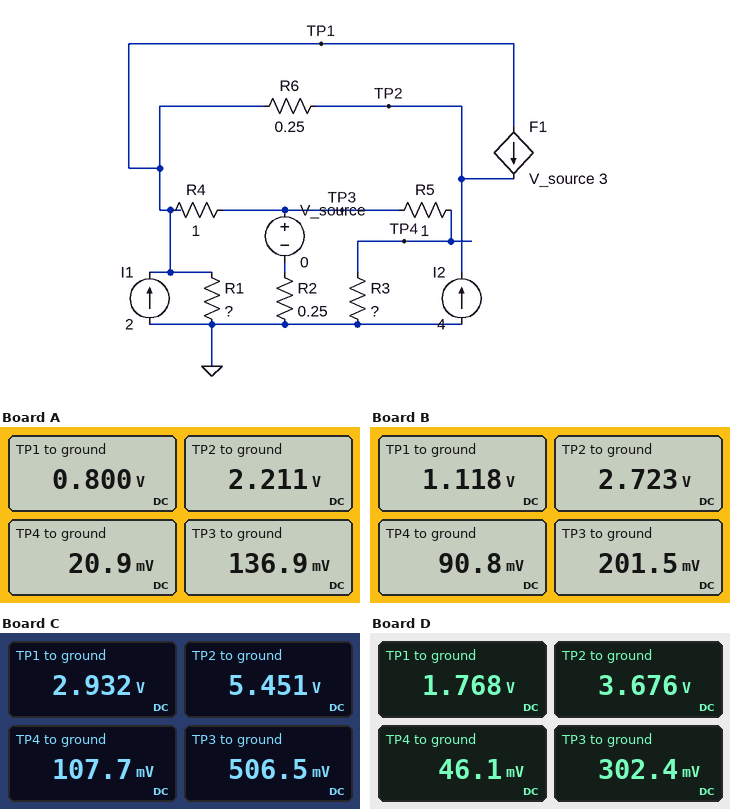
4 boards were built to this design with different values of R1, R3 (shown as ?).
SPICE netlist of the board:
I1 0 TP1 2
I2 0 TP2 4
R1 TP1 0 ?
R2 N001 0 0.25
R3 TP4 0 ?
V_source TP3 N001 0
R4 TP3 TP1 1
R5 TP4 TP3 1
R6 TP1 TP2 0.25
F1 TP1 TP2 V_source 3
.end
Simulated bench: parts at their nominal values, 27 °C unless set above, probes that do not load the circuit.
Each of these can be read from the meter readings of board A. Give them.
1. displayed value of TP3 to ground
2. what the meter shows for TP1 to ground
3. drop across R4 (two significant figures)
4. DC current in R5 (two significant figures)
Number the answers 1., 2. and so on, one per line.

1. 136.9 mV
2. 0.800 V
3. 660 mV
4. 120 mA
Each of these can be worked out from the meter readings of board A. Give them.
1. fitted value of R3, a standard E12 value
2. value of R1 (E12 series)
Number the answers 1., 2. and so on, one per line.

1. 0.18 Ω
2. 0.15 Ω
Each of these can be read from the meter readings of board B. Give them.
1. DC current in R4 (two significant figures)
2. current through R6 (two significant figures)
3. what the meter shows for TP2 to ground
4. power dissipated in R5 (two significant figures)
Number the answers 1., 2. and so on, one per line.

1. 920 mA
2. 6.4 A
3. 2.723 V
4. 12 mW
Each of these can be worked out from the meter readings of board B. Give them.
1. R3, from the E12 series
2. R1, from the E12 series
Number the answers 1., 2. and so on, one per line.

1. 0.82 Ω
2. 0.22 Ω
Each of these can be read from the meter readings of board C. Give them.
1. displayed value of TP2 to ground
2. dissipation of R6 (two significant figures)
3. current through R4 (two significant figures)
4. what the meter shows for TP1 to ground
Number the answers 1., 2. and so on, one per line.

1. 5.451 V
2. 25 W
3. 2.4 A
4. 2.932 V
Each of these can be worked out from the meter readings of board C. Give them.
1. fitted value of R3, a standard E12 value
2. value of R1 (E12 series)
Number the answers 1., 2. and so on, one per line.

1. 0.27 Ω
2. 0.82 Ω
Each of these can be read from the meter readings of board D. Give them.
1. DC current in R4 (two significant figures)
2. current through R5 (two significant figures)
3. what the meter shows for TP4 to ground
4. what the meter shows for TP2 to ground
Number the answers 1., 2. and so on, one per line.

1. 1.5 A
2. 260 mA
3. 46.1 mV
4. 3.676 V
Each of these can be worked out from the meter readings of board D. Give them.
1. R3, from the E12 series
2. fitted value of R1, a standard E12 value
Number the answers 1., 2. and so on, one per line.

1. 0.18 Ω
2. 0.39 Ω
